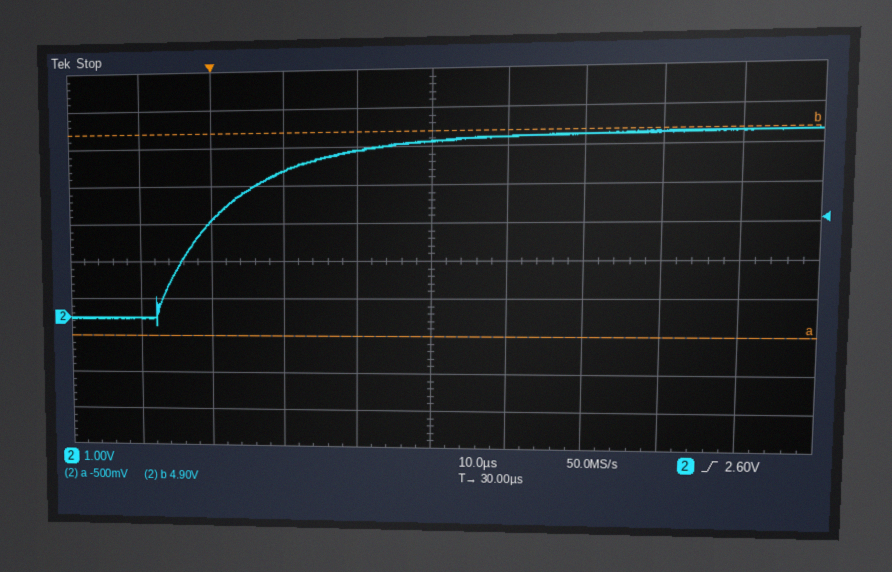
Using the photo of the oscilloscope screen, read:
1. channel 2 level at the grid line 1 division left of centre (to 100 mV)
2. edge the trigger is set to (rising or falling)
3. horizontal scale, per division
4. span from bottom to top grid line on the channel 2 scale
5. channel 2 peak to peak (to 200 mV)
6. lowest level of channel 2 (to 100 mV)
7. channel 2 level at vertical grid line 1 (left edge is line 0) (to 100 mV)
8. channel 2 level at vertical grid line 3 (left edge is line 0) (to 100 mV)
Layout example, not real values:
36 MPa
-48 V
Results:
4.4 V
rising
10 µs
10 V
5.0 V
-200 mV
0.0 V
3.9 V
